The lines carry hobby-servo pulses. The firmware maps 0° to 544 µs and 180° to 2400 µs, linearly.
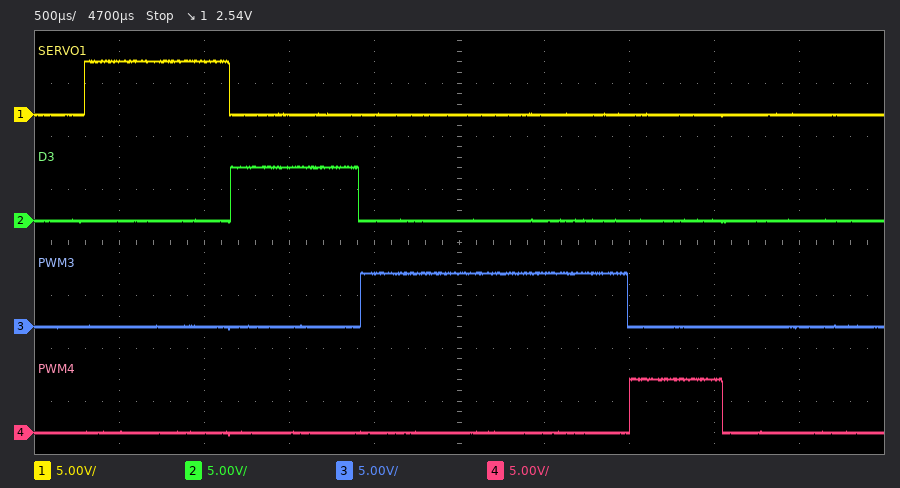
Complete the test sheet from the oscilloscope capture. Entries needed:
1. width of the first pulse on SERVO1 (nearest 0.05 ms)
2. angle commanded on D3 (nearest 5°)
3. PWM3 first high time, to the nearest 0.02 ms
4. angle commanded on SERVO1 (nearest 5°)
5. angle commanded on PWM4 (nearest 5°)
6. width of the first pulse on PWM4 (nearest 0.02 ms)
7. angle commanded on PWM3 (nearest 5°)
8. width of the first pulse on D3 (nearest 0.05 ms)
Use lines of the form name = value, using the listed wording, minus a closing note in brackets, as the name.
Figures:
width of the first pulse on SERVO1 = 0.85 ms
angle commanded on D3 = 20°
PWM3 first high time, to the nearest 0.02 ms = 1.58 ms
angle commanded on SERVO1 = 30°
angle commanded on PWM4 = 0°
width of the first pulse on PWM4 = 0.54 ms
angle commanded on PWM3 = 100°
width of the first pulse on D3 = 0.75 ms
